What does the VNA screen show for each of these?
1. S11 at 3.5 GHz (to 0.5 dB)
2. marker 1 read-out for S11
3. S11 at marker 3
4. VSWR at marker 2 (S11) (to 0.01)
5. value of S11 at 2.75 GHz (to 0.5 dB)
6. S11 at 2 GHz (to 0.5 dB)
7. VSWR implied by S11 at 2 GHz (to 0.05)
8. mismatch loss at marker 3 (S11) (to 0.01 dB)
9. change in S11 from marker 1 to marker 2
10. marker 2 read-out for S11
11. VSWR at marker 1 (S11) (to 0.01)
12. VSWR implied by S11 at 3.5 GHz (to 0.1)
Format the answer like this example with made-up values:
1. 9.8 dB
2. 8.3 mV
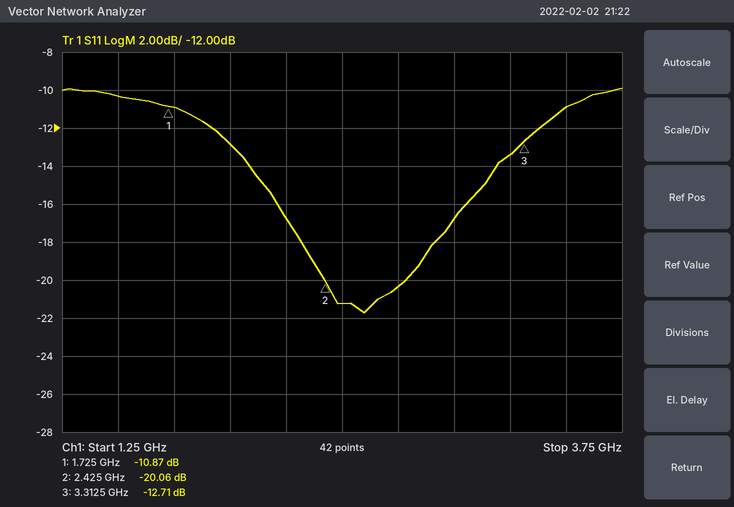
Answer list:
1. -11.0 dB
2. -10.87 dB
3. -12.71 dB
4. 1.22
5. -20.5 dB
6. -13.0 dB
7. 1.60
8. 0.24 dB
9. -9.19 dB
10. -20.06 dB
11. 1.80
12. 1.8
